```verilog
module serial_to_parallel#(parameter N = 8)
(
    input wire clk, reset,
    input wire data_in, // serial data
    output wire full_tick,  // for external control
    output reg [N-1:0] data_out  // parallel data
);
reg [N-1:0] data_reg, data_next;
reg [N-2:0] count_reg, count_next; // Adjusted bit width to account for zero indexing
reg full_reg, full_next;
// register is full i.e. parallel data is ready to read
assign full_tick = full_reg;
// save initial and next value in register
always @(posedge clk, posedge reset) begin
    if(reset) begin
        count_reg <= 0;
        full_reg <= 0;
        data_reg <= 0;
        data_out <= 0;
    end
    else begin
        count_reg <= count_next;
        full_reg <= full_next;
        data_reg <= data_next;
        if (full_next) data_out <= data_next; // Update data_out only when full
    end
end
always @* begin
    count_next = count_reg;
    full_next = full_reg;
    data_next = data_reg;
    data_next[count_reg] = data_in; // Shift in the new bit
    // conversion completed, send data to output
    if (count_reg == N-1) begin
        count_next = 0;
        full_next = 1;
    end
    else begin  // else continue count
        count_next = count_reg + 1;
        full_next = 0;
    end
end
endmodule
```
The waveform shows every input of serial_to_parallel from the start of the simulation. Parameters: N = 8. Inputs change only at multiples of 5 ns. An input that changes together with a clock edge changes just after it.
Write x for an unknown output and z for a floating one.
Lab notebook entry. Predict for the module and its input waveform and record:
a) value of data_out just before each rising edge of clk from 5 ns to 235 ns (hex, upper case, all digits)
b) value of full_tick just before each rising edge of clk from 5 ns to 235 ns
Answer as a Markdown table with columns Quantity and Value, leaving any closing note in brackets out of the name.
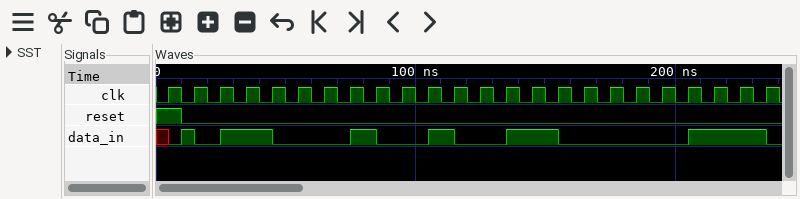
| Quantity | Value |
|---|---|
| value of data_out just before each rising edge of clk from 5 ns to 235 ns | 00, 00, 00, 00, 00, 00, 00, 00, 00, 8D, 8D, 8D, 8D, 8D, 8D, 8D, 8D, 64, 64, 64, 64, 64, 64, 64 |
| value of full_tick just before each rising edge of clk from 5 ns to 235 ns | 0 0 0 0 0 0 0 0 0 1 0 0 0 0 0 0 0 1 0 0 0 0 0 0 |
